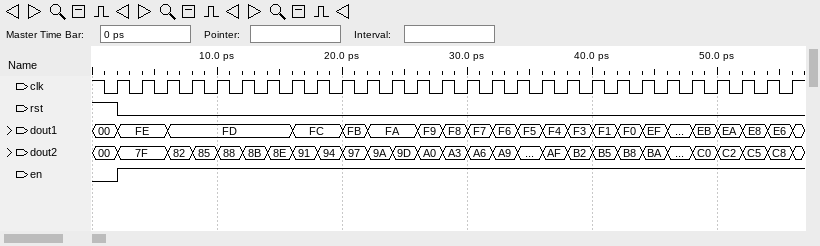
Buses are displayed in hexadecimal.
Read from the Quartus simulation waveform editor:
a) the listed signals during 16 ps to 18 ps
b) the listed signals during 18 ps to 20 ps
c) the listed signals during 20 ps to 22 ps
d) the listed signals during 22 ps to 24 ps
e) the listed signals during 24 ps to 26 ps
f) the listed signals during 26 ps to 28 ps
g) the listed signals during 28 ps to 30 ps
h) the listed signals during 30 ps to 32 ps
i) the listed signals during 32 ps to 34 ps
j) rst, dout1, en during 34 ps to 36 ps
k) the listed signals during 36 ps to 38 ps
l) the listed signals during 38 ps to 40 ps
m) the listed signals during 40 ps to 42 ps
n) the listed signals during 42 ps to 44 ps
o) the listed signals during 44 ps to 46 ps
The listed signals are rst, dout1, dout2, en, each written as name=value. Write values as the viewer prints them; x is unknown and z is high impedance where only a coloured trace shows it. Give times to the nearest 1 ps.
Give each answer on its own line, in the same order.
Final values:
rst=0, dout1=FC, dout2=91, en=1
rst=0, dout1=FC, dout2=94, en=1
rst=0, dout1=FB, dout2=97, en=1
rst=0, dout1=FA, dout2=9A, en=1
rst=0, dout1=FA, dout2=9D, en=1
rst=0, dout1=F9, dout2=A0, en=1
rst=0, dout1=F8, dout2=A3, en=1
rst=0, dout1=F7, dout2=A6, en=1
rst=0, dout1=F6, dout2=A9, en=1
rst=0, dout1=F5, en=1
rst=0, dout1=F4, dout2=AF, en=1
rst=0, dout1=F3, dout2=B2, en=1
rst=0, dout1=F1, dout2=B5, en=1
rst=0, dout1=F0, dout2=B8, en=1
rst=0, dout1=EF, dout2=BA, en=1
